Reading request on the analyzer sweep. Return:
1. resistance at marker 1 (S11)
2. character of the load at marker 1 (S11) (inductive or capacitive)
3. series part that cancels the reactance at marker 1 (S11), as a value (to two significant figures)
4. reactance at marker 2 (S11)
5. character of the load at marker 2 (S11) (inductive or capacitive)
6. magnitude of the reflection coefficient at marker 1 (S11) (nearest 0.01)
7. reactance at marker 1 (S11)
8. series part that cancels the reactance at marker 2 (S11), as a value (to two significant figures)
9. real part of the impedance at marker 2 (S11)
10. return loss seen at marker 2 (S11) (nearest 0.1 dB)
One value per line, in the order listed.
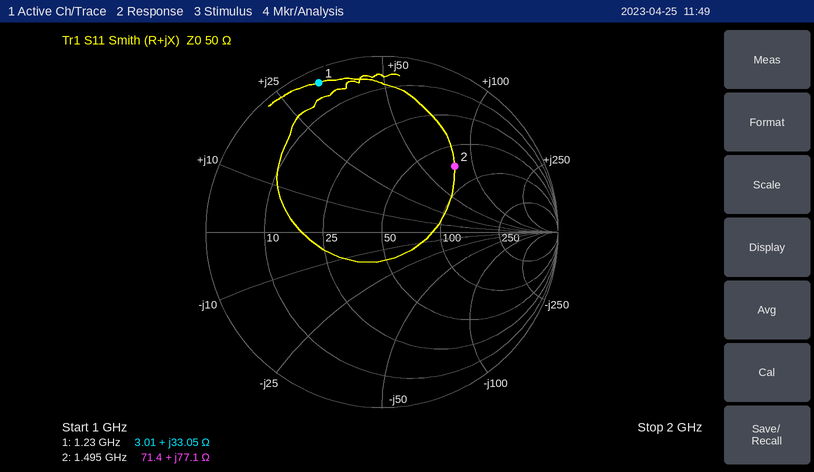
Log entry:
3.01 Ω
inductive
3.9 pF
+77.1 Ω
inductive
0.92
+33.05 Ω
1.4 pF
71.4 Ω
5.1 dB
